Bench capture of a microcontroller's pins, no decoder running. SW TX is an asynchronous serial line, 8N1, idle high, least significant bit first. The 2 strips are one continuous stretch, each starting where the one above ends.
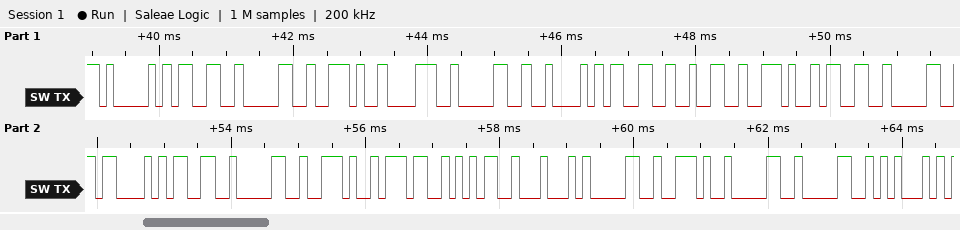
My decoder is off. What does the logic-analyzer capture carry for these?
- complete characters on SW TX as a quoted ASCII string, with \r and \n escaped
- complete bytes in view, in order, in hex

"A30.80B32.30C30.75D0.00E"
0x41 0x33 0x30 0x2E 0x38 0x30 0x42 0x33 0x32 0x2E 0x33 0x30 0x43 0x33 0x30 0x2E 0x37 0x35 0x44 0x30 0x2E 0x30 0x30 0x45
